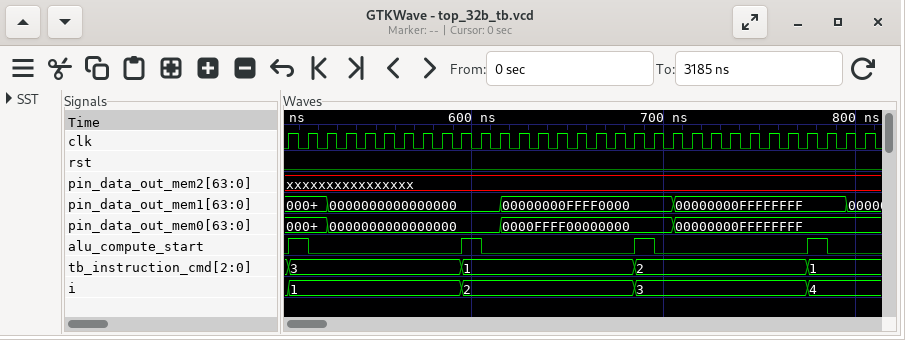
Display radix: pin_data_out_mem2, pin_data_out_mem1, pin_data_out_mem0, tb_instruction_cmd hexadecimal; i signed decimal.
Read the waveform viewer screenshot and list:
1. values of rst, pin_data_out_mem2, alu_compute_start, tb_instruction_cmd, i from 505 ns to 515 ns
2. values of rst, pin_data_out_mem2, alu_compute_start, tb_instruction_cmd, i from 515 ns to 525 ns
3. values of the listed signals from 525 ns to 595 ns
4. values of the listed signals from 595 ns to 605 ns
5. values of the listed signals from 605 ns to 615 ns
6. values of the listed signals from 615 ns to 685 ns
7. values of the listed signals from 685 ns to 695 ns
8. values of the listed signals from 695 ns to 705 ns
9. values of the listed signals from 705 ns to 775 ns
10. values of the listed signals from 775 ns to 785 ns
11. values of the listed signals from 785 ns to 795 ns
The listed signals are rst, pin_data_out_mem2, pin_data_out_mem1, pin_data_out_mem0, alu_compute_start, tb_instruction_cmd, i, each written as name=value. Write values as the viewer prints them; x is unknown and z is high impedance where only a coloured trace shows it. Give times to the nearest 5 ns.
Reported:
rst=0, pin_data_out_mem2=xxxxxxxxxxxxxxxx, alu_compute_start=1, tb_instruction_cmd=3, i=1
rst=0, pin_data_out_mem2=xxxxxxxxxxxxxxxx, alu_compute_start=0, tb_instruction_cmd=3, i=1
rst=0, pin_data_out_mem2=xxxxxxxxxxxxxxxx, pin_data_out_mem1=0000000000000000, pin_data_out_mem0=0000000000000000, alu_compute_start=0, tb_instruction_cmd=3, i=1
rst=0, pin_data_out_mem2=xxxxxxxxxxxxxxxx, pin_data_out_mem1=0000000000000000, pin_data_out_mem0=0000000000000000, alu_compute_start=1, tb_instruction_cmd=1, i=2
rst=0, pin_data_out_mem2=xxxxxxxxxxxxxxxx, pin_data_out_mem1=0000000000000000, pin_data_out_mem0=0000000000000000, alu_compute_start=0, tb_instruction_cmd=1, i=2
rst=0, pin_data_out_mem2=xxxxxxxxxxxxxxxx, pin_data_out_mem1=00000000FFFF0000, pin_data_out_mem0=0000FFFF00000000, alu_compute_start=0, tb_instruction_cmd=1, i=2
rst=0, pin_data_out_mem2=xxxxxxxxxxxxxxxx, pin_data_out_mem1=00000000FFFF0000, pin_data_out_mem0=0000FFFF00000000, alu_compute_start=1, tb_instruction_cmd=2, i=3
rst=0, pin_data_out_mem2=xxxxxxxxxxxxxxxx, pin_data_out_mem1=00000000FFFF0000, pin_data_out_mem0=0000FFFF00000000, alu_compute_start=0, tb_instruction_cmd=2, i=3
rst=0, pin_data_out_mem2=xxxxxxxxxxxxxxxx, pin_data_out_mem1=00000000FFFFFFFF, pin_data_out_mem0=00000000FFFFFFFF, alu_compute_start=0, tb_instruction_cmd=2, i=3
rst=0, pin_data_out_mem2=xxxxxxxxxxxxxxxx, pin_data_out_mem1=00000000FFFFFFFF, pin_data_out_mem0=00000000FFFFFFFF, alu_compute_start=1, tb_instruction_cmd=1, i=4
rst=0, pin_data_out_mem2=xxxxxxxxxxxxxxxx, pin_data_out_mem1=00000000FFFFFFFF, pin_data_out_mem0=00000000FFFFFFFF, alu_compute_start=0, tb_instruction_cmd=1, i=4
